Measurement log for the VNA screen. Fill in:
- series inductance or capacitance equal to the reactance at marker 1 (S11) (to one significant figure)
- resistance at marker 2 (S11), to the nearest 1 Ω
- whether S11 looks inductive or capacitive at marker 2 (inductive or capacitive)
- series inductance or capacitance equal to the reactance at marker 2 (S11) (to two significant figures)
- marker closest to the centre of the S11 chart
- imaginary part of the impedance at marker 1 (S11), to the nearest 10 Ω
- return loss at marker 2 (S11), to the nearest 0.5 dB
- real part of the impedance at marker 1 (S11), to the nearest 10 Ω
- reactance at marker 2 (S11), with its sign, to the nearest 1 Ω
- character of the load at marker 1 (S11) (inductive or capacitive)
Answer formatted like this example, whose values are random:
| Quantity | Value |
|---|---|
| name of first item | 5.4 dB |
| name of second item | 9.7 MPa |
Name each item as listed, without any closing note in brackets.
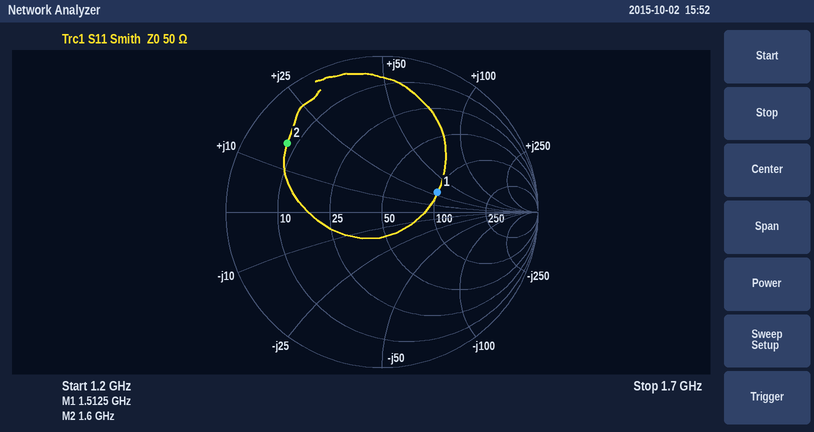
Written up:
| Quantity | Value |
|---|---|
| series inductance or capacitance equal to the reactance at marker 1 (S11) | 3 nH |
| resistance at marker 2 (S11), to the nearest 1 Ω | 8 Ω |
| whether S11 looks inductive or capacitive at marker 2 | inductive |
| series inductance or capacitance equal to the reactance at marker 2 (S11) | 1.6 nH |
| marker closest to the centre of the S11 chart | marker 1 |
| imaginary part of the impedance at marker 1 (S11), to the nearest 10 Ω | +30 Ω |
| return loss at marker 2 (S11), to the nearest 0.5 dB | 2.5 dB |
| real part of the impedance at marker 1 (S11), to the nearest 10 Ω | 100 Ω |
| reactance at marker 2 (S11), with its sign, to the nearest 1 Ω | +16 Ω |
| character of the load at marker 1 (S11) | inductive |
